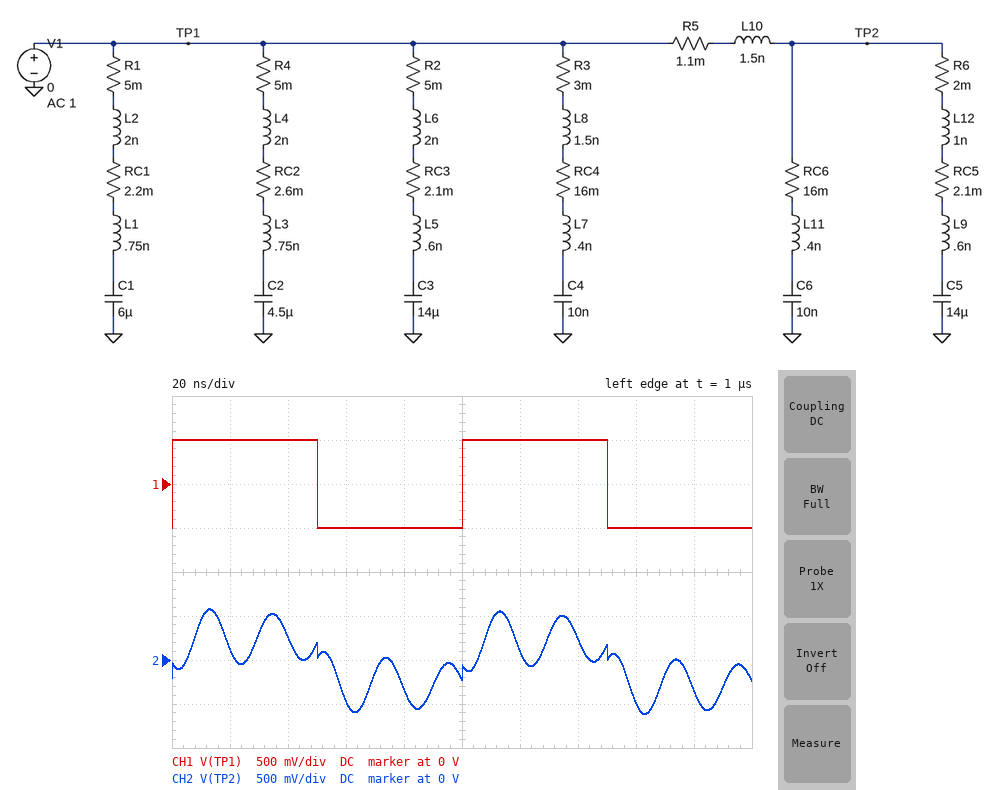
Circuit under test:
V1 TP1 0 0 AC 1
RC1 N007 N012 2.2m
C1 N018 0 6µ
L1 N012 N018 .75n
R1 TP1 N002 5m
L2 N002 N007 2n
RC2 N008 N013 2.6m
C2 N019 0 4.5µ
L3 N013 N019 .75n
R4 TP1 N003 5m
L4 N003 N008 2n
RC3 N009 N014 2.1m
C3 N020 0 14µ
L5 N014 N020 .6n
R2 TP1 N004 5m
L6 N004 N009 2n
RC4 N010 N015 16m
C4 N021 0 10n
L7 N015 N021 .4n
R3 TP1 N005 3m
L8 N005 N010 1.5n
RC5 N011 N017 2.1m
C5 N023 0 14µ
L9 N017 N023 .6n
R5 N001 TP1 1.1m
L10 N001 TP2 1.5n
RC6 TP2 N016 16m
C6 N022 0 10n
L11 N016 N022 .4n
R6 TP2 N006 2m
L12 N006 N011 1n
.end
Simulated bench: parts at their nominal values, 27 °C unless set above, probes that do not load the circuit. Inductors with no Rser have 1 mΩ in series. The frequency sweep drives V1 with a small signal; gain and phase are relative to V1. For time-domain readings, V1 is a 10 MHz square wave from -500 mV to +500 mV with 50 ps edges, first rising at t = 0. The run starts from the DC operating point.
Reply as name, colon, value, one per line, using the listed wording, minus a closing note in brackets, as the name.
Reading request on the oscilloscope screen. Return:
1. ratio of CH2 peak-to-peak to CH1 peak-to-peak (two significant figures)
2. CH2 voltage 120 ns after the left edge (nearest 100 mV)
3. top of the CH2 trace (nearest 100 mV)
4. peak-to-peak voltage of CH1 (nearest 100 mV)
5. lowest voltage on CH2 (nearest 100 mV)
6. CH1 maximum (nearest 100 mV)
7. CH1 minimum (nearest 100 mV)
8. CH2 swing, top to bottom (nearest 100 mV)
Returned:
ratio of CH2 peak-to-peak to CH1 peak-to-peak: 1.2
CH2 voltage 120 ns after the left edge: 100 mV
top of the CH2 trace: 600 mV
peak-to-peak voltage of CH1: 1.0 V
lowest voltage on CH2: -600 mV
CH1 maximum: 500 mV
CH1 minimum: -500 mV
CH2 swing, top to bottom: 1.2 V
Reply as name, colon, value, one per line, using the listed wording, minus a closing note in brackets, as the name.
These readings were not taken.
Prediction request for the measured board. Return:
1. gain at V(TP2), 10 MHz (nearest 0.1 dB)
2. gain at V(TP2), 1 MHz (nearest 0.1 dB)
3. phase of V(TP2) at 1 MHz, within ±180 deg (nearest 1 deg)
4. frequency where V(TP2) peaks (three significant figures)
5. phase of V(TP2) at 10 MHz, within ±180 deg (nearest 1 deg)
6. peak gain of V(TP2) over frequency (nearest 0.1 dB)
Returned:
gain at V(TP2), 10 MHz: -5.5 dB
gain at V(TP2), 1 MHz: -5.3 dB
phase of V(TP2) at 1 MHz, within ±180 deg: -57 deg
frequency where V(TP2) peaks: 46.4 MHz
phase of V(TP2) at 10 MHz, within ±180 deg: -1 deg
peak gain of V(TP2) over frequency: 15.8 dB
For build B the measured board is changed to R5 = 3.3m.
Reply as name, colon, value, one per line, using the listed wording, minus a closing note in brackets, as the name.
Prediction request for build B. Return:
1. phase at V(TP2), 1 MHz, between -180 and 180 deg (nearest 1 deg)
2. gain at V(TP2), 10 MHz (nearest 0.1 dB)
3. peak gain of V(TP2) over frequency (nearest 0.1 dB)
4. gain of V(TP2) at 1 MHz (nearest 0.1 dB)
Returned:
phase at V(TP2), 1 MHz, between -180 and 180 deg: -50 deg
gain at V(TP2), 10 MHz: -5.5 dB
peak gain of V(TP2) over frequency: 15.5 dB
gain of V(TP2) at 1 MHz: -6.5 dB
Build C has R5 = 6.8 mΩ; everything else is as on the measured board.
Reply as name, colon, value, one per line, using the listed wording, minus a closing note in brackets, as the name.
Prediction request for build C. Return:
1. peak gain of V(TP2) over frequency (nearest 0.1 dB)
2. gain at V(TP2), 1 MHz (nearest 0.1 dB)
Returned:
peak gain of V(TP2) over frequency: 15.1 dB
gain at V(TP2), 1 MHz: -8.2 dB
